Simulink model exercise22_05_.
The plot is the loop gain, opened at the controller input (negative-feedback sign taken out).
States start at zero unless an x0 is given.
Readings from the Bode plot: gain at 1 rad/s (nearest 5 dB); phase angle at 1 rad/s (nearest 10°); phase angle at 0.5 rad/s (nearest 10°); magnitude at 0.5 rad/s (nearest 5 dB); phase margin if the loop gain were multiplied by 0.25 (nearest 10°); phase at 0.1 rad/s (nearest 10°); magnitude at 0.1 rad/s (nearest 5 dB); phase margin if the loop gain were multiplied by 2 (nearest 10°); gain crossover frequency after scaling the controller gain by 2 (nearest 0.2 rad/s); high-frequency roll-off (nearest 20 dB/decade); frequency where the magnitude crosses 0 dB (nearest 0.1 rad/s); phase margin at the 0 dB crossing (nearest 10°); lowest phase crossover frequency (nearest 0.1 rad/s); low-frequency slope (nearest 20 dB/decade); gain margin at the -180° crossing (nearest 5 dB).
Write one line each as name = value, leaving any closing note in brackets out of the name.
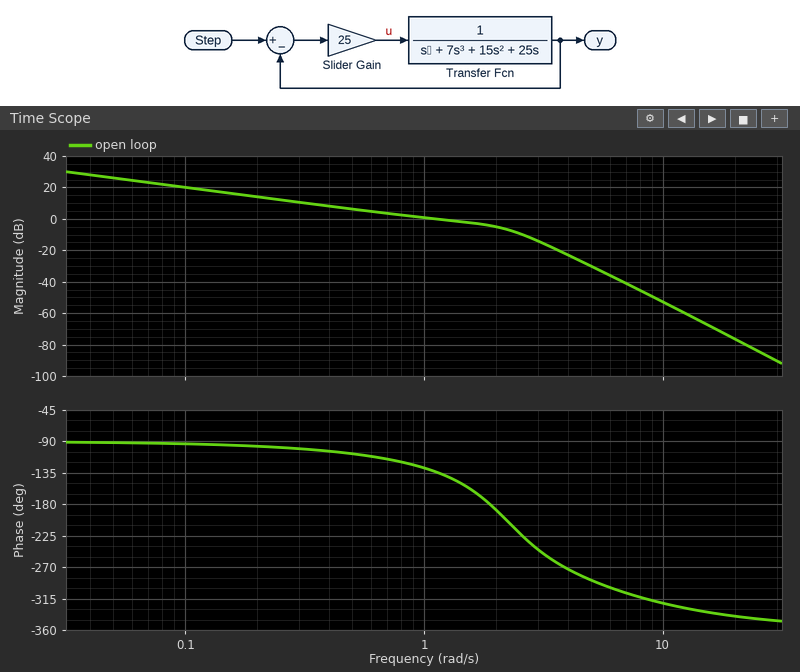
gain at 1 rad/s = 0 dB
phase angle at 1 rad/s = -130°
phase angle at 0.5 rad/s = -110°
magnitude at 0.5 rad/s = 5 dB
phase margin if the loop gain were multiplied by 0.25 = 80°
phase at 0.1 rad/s = -90°
magnitude at 0.1 rad/s = 20 dB
phase margin if the loop gain were multiplied by 2 = -20°
gain crossover frequency after scaling the controller gain by 2 = 2.2 rad/s
high-frequency roll-off = -80 dB/decade
frequency where the magnitude crosses 0 dB = 1.1 rad/s
phase margin at the 0 dB crossing = 50°
lowest phase crossover frequency = 1.9 rad/s
low-frequency slope = -20 dB/decade
gain margin at the -180° crossing = 5 dB
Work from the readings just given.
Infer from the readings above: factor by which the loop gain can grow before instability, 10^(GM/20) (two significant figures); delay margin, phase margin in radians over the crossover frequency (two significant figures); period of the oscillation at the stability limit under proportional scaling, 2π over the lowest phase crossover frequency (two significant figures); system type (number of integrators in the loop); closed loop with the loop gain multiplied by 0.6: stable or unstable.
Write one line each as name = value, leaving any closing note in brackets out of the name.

factor by which the loop gain can grow before instability, 10^(GM/20) = 1.8
delay margin, phase margin in radians over the crossover frequency = 0.79 s
period of the oscillation at the stability limit under proportional scaling, 2π over the lowest phase crossover frequency = 3.3 s
system type = 1
closed loop with the loop gain multiplied by 0.6: stable or unstable = stable
